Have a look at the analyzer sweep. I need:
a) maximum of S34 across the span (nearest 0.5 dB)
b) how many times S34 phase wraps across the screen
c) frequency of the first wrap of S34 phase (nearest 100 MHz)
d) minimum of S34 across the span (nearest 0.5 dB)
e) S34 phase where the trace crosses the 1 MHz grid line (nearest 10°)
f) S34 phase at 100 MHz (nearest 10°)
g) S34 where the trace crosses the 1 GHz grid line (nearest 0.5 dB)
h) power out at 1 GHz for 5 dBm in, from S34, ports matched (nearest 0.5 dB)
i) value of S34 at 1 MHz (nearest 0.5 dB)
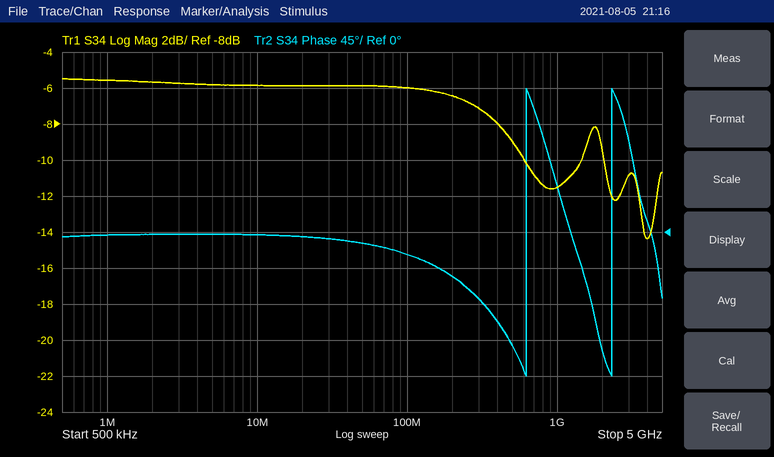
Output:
-5.5 dB
2
600 MHz
-14.5 dB
0°
-30°
-11.5 dB
-6.5 dBm
-5.5 dB
